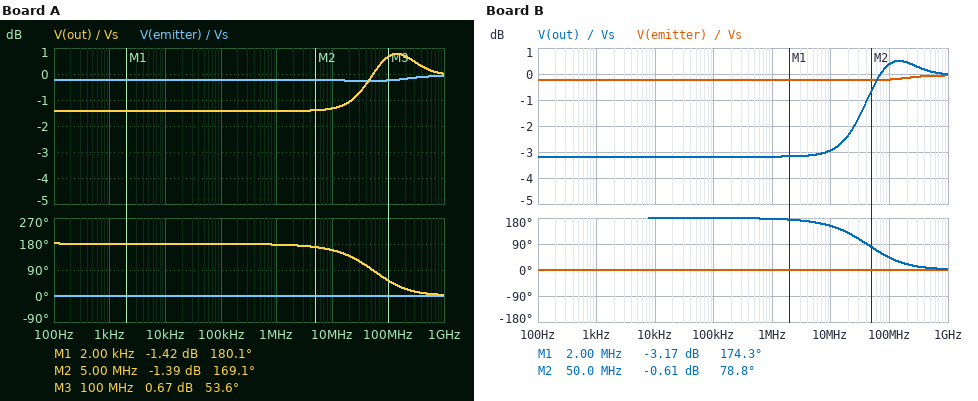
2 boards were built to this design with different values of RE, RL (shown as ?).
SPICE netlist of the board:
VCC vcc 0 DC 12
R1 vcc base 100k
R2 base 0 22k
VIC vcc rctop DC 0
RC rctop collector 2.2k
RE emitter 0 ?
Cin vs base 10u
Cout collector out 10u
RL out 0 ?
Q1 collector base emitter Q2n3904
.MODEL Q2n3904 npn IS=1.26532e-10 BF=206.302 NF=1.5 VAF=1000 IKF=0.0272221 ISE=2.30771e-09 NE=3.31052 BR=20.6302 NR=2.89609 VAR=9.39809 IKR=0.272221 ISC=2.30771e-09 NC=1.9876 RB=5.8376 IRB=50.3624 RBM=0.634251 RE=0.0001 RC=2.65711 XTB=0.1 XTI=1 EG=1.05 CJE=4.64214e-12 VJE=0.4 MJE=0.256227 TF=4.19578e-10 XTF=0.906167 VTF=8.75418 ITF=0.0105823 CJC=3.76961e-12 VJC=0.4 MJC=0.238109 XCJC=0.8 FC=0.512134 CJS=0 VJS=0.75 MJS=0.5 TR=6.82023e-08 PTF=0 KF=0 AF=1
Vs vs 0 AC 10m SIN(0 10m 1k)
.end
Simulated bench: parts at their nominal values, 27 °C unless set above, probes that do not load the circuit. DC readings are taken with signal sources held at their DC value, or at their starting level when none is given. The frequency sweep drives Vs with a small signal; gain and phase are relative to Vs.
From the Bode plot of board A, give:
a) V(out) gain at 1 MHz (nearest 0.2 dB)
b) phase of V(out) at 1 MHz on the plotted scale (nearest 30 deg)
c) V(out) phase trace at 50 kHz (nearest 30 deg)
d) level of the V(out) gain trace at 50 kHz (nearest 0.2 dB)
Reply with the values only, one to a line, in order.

-1.4 dB
180 deg
180 deg
-1.4 dB
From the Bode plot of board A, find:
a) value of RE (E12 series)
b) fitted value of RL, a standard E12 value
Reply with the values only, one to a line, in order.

1.5 kΩ
3.3 kΩ
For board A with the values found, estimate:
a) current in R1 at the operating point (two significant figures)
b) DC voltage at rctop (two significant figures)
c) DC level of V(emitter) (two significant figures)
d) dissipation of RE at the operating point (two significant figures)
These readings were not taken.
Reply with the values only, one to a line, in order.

100 µA
12 V
1.4 V
1.3 mW
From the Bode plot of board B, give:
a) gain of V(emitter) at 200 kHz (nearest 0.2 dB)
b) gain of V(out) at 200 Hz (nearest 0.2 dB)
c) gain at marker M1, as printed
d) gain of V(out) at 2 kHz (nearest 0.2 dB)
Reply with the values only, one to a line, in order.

-0.2 dB
-3.2 dB
-3.17 dB
-3.2 dB
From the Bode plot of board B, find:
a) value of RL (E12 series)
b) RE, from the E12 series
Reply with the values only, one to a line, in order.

5.6 kΩ
2.2 kΩ
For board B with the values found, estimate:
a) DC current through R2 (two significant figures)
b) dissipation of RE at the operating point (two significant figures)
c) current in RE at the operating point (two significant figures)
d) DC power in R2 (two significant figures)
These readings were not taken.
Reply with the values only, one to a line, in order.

93 µA
960 µW
660 µA
190 µW
